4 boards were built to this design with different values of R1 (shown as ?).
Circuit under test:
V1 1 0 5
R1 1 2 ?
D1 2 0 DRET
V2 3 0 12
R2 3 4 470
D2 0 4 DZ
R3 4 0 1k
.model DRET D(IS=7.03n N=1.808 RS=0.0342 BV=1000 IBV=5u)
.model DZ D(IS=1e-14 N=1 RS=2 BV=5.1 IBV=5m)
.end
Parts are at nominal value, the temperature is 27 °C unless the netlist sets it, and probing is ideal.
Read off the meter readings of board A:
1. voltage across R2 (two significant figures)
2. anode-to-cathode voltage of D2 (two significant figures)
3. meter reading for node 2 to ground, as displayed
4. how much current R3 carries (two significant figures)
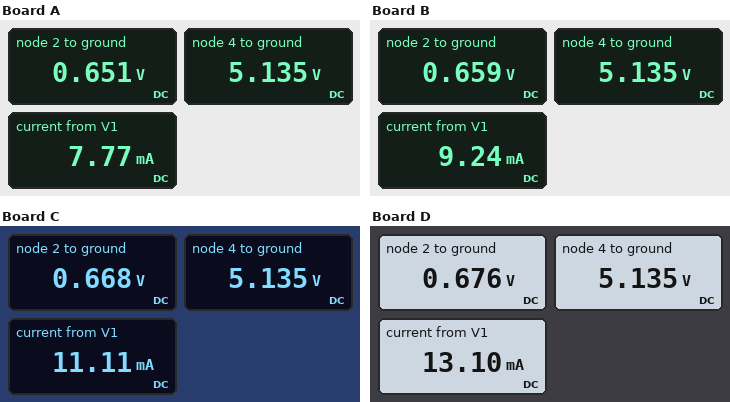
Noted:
6.9 V
-5.1 V
0.651 V
5.1 mA
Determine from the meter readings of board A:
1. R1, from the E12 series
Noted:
560 Ω
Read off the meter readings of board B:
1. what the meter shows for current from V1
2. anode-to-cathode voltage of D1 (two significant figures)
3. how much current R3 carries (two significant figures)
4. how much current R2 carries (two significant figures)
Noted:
9.24 mA
660 mV
5.1 mA
15 mA
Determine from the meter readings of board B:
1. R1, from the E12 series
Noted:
470 Ω
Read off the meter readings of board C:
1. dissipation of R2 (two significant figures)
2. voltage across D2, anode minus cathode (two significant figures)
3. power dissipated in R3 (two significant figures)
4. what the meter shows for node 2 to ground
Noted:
100 mW
-5.1 V
26 mW
0.668 V
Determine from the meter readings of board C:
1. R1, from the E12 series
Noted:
390 Ω
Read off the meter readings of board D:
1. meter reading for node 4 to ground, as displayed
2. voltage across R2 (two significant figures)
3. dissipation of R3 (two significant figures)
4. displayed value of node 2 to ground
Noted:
5.135 V
6.9 V
26 mW
0.676 V
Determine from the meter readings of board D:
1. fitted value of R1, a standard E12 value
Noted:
330 Ω
